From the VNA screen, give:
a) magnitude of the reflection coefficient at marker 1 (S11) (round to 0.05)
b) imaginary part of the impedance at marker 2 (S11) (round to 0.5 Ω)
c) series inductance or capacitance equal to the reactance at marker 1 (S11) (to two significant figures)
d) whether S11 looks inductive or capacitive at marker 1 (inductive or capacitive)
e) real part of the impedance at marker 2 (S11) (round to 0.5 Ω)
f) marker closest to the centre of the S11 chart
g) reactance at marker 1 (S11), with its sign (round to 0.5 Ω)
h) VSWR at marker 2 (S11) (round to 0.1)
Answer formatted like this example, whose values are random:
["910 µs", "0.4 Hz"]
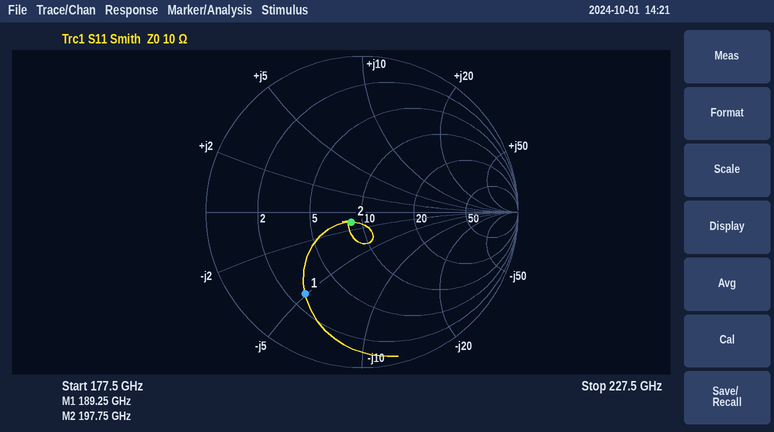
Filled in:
["0.65", "-1.0 Ω", "170 fF", "capacitive", "8.5 Ω", "marker 2", "-5.0 Ω", "1.2"]
